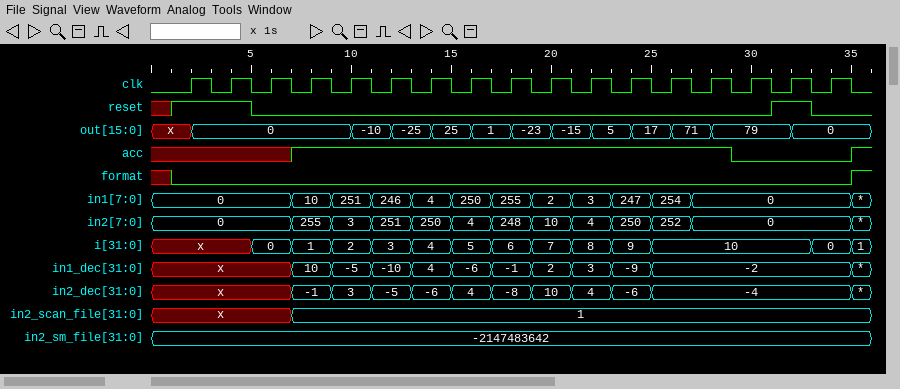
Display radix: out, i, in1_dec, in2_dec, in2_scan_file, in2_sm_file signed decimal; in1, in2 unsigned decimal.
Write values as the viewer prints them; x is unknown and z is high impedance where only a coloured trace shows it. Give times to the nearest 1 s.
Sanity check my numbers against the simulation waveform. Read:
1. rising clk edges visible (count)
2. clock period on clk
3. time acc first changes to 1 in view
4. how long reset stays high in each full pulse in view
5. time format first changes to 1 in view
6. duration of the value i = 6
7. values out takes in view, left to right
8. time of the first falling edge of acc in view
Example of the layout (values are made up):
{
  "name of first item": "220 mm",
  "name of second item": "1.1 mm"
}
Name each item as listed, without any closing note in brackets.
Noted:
{
  "rising clk edges visible": "17",
  "clock period on clk": "2 s",
  "time acc first changes to 1 in view": "7 s",
  "how long reset stays high in each full pulse in view": "2 s",
  "time format first changes to 1 in view": "35 s",
  "duration of the value i = 6": "2 s",
  "values out takes in view, left to right": "x, 0, -10, -25, 25, 1, -23, -15, 5, 17, 71, 79, 0",
  "time of the first falling edge of acc in view": "29 s"
}
